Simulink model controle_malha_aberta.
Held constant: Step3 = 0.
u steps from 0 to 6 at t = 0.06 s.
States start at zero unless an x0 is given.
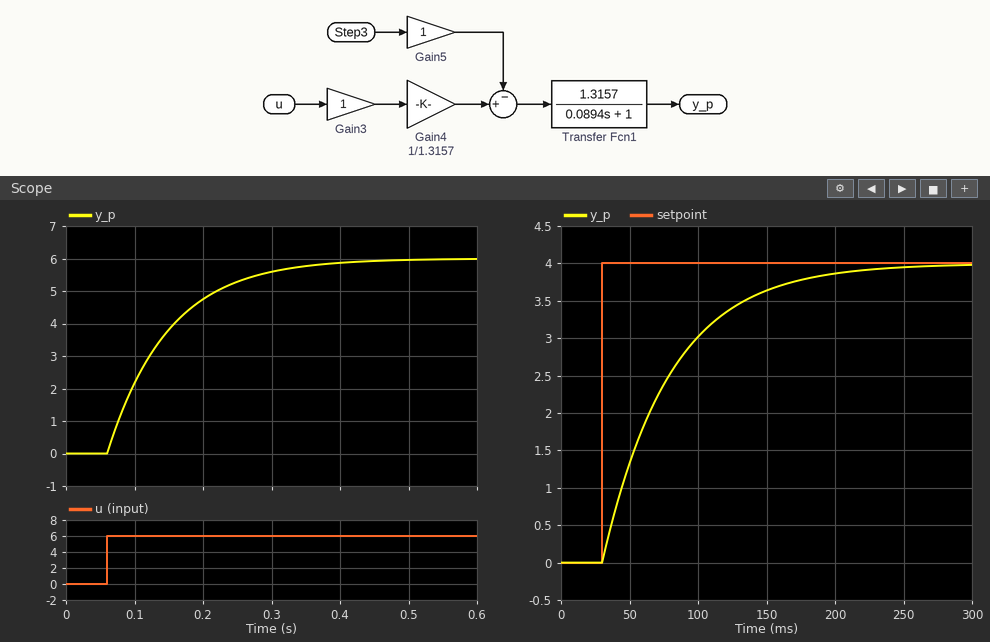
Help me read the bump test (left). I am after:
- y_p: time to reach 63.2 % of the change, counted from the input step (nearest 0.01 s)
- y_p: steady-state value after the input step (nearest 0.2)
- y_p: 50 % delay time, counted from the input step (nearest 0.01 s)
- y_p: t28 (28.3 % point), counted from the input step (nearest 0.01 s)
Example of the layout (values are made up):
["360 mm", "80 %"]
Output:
["0.09 s", "6.0", "0.06 s", "0.03 s"]
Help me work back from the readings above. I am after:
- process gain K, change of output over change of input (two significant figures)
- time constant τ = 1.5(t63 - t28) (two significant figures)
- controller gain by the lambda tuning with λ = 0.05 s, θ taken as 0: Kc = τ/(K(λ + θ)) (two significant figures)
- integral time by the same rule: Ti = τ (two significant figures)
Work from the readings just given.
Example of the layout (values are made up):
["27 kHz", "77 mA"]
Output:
["1.0", "0.090 s", "1.8", "0.090 s"]
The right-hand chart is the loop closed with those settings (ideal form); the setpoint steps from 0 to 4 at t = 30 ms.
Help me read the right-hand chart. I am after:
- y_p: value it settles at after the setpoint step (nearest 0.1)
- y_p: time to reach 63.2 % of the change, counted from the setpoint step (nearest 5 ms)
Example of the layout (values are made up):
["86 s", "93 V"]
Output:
["4.0", "50 ms"]
